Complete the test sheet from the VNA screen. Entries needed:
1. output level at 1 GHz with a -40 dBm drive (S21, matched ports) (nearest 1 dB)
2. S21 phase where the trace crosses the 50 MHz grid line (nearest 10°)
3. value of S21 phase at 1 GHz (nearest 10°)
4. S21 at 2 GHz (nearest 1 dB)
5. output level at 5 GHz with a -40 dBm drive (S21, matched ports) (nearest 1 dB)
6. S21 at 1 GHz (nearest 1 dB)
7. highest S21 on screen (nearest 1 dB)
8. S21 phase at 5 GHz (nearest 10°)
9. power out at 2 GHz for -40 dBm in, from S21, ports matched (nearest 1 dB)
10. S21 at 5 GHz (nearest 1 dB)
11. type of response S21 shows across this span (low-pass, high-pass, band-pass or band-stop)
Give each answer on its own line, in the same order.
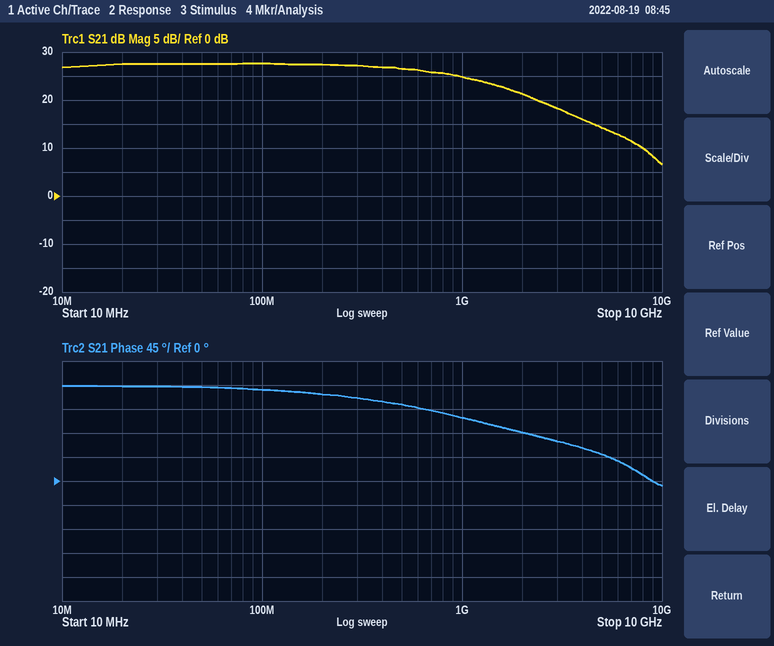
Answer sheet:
-15 dBm
180°
120°
21 dB
-26 dBm
25 dB
28 dB
50°
-19 dBm
14 dB
low-pass
